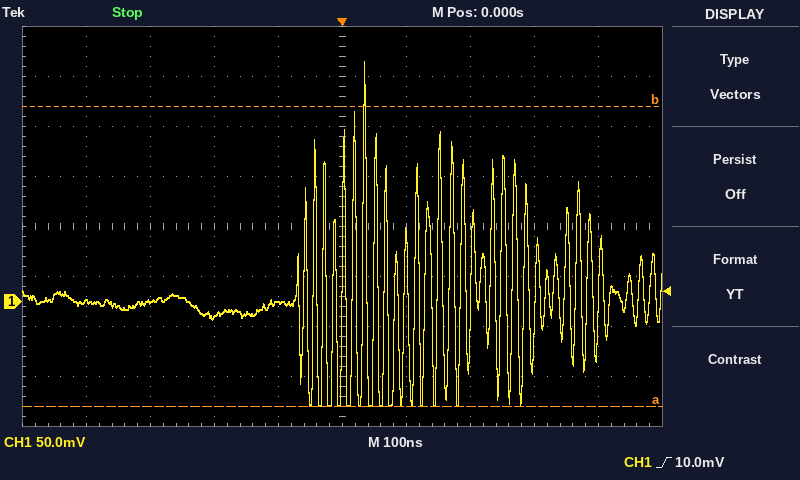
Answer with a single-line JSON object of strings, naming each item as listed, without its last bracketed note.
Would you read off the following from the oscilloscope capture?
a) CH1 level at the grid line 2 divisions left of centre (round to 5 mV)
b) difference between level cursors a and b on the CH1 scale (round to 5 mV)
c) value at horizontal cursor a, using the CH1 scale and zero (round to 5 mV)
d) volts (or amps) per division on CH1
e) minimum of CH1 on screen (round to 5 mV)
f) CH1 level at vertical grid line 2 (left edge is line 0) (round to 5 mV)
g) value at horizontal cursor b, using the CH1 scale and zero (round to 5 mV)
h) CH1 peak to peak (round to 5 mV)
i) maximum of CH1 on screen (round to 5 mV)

{"CH1 level at the grid line 2 divisions left of centre": "-15 mV", "difference between level cursors a and b on the CH1 scale": "300 mV", "value at horizontal cursor a, using the CH1 scale and zero": "-105 mV", "volts (or amps) per division on CH1": "50 mV", "minimum of CH1 on screen": "-105 mV", "CH1 level at vertical grid line 2 (left edge is line 0)": "0 mV", "value at horizontal cursor b, using the CH1 scale and zero": "195 mV", "CH1 peak to peak": "345 mV", "maximum of CH1 on screen": "240 mV"}
